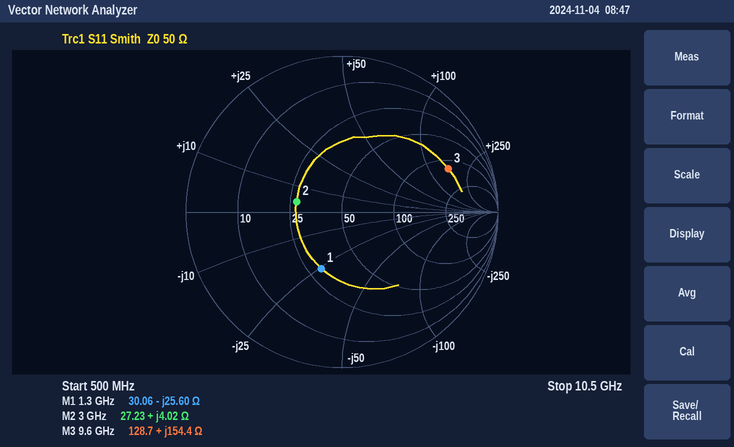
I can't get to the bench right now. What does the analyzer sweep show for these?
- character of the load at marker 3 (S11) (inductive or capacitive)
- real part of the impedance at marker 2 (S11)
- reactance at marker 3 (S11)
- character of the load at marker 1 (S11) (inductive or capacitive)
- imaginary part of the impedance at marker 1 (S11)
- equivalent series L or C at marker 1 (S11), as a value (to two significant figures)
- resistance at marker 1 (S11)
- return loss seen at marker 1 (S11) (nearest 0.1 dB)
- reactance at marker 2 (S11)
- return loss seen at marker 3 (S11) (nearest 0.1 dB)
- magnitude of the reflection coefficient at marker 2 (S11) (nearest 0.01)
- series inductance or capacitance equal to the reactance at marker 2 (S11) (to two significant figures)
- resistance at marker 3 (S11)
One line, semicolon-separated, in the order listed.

inductive; 27.23 Ω; +154.4 Ω; capacitive; -25.60 Ω; 4.8 pF; 30.06 Ω; 8.3 dB; +4.02 Ω; 2.7 dB; 0.30; 210 pH; 128.7 Ω
